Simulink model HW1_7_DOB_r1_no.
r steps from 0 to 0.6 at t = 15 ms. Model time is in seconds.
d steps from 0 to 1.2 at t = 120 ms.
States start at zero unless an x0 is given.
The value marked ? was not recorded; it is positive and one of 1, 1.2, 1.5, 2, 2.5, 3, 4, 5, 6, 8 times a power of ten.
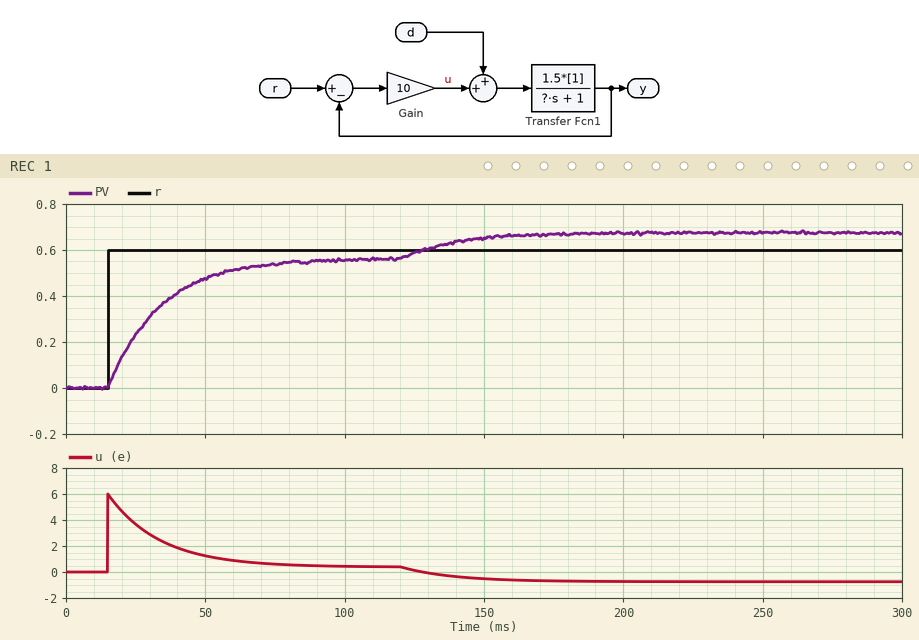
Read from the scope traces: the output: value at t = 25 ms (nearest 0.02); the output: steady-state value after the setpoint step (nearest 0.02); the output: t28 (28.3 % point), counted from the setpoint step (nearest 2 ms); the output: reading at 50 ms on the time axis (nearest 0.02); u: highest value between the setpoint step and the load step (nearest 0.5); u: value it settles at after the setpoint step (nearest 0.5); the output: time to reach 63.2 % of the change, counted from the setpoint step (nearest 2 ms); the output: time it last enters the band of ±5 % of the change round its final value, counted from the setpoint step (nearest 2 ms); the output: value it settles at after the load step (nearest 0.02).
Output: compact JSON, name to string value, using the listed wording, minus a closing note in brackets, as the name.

{"the output: value at t = 25 ms": "0.24", "the output: steady-state value after the setpoint step": "0.56", "the output: t28 (28.3 % point), counted from the setpoint step": "6 ms", "the output: reading at 50 ms on the time axis": "0.48", "u: highest value between the setpoint step and the load step": "6.0", "u: value it settles at after the setpoint step": "0.5", "the output: time to reach 63.2 % of the change, counted from the setpoint step": "18 ms", "the output: time it last enters the band of ±5 % of the change round its final value, counted from the setpoint step": "56 ms", "the output: value it settles at after the load step": "0.68"}
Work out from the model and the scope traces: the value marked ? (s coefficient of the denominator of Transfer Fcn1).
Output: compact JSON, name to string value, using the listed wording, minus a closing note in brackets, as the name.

{"the value marked ?": "0.3"}
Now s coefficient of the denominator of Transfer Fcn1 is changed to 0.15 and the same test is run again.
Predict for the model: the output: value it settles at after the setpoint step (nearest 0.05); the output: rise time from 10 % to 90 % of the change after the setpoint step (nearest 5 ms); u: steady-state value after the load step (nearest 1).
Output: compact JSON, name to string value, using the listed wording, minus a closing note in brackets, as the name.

{"the output: value it settles at after the setpoint step": "0.55", "the output: rise time from 10 % to 90 % of the change after the setpoint step": "20 ms", "u: steady-state value after the load step": "-1"}
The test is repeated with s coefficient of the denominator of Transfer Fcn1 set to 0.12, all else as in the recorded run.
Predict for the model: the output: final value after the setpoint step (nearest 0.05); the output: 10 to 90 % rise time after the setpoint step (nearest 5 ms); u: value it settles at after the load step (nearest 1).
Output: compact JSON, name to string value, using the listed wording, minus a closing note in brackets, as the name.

{"the output: final value after the setpoint step": "0.55", "the output: 10 to 90 % rise time after the setpoint step": "15 ms", "u: value it settles at after the load step": "-1"}
